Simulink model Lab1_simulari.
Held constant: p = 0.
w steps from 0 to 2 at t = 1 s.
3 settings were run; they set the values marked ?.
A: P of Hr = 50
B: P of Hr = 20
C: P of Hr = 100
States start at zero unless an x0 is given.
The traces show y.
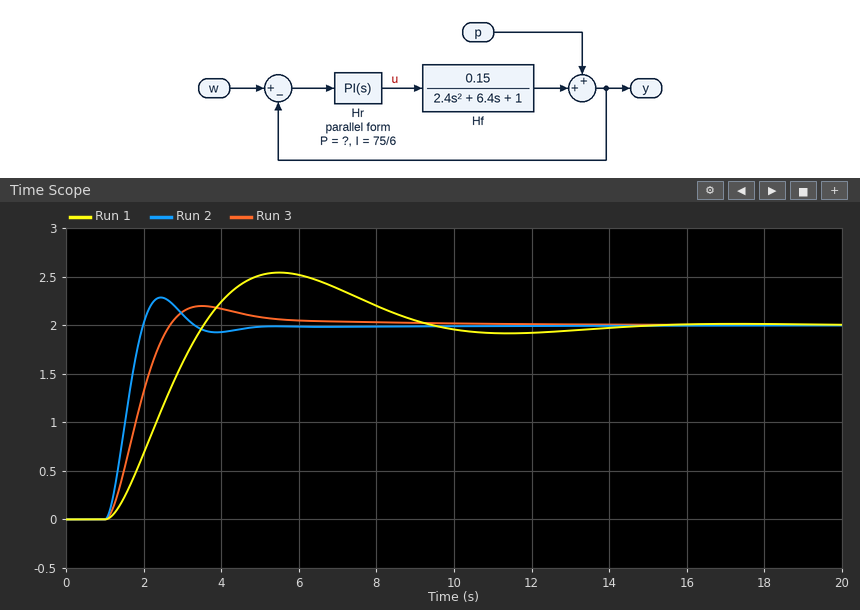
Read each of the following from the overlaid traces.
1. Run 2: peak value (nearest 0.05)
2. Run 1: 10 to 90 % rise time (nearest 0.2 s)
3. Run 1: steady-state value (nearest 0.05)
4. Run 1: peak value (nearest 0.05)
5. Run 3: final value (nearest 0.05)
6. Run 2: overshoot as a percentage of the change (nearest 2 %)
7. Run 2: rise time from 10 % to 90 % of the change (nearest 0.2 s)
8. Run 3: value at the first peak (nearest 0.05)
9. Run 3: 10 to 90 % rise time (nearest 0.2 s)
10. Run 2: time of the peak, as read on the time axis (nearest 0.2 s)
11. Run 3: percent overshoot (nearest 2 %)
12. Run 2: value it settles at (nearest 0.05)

2.30
1.8 s
2.00
2.55
2.00
14 %
0.6 s
2.20
1.2 s
2.4 s
10 %
2.00
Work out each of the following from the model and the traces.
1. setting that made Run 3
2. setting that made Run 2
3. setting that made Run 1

A
C
B
